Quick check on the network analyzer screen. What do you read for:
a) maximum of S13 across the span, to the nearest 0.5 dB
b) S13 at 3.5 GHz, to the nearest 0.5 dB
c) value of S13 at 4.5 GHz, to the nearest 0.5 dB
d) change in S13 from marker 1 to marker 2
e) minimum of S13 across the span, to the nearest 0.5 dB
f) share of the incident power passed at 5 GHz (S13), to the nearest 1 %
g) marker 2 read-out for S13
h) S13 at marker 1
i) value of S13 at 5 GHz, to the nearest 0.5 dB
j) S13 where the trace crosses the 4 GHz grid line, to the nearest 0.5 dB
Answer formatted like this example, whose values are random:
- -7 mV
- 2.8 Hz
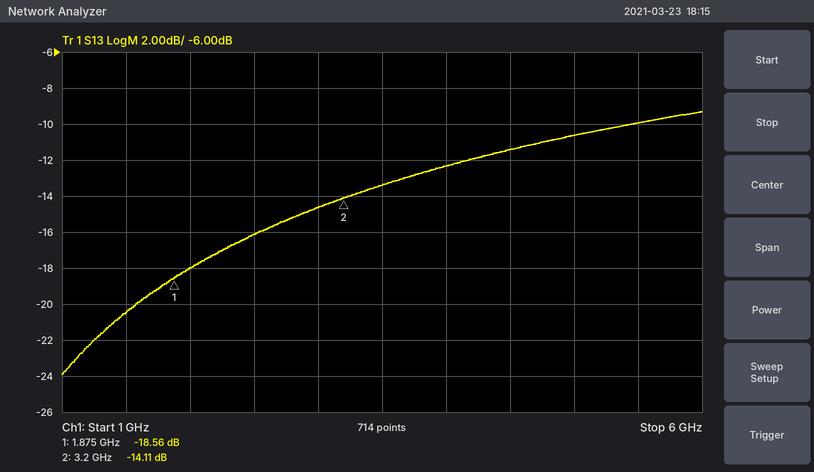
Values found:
- -9.5 dB
- -13.5 dB
- -11.5 dB
- 4.45 dB
- -24.0 dB
- 9 %
- -14.11 dB
- -18.56 dB
- -10.5 dB
- -12.5 dB
